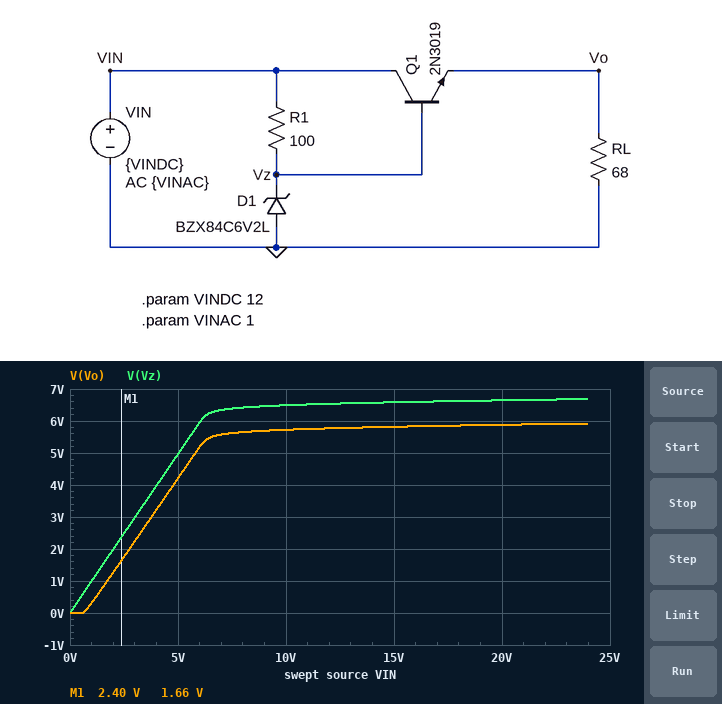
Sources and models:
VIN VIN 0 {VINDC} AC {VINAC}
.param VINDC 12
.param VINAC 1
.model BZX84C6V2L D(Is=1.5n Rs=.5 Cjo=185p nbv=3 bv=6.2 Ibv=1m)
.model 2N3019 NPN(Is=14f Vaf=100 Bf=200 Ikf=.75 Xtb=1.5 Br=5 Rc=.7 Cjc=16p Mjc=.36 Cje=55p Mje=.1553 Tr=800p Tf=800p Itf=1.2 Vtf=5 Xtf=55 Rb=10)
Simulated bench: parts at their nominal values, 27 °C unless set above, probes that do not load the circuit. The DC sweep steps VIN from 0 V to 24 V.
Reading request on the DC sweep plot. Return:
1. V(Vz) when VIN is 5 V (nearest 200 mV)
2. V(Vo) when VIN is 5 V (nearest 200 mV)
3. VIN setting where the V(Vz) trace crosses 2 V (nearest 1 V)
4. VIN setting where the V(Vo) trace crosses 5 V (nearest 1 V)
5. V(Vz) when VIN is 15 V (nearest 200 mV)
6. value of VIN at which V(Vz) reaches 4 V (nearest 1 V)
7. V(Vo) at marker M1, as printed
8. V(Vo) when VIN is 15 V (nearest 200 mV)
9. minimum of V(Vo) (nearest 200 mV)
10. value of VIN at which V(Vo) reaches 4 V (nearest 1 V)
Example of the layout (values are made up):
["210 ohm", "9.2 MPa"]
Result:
["5.0 V", "4.2 V", "2 V", "6 V", "6.6 V", "4 V", "1.66 V", "5.8 V", "0 V", "5 V"]
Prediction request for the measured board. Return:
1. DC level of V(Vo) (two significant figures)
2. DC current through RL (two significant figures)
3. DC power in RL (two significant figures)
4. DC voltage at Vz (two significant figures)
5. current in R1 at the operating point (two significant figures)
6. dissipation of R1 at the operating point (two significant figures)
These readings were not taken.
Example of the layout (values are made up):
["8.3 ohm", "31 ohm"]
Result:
["5.8 V", "85 mA", "490 mW", "6.5 V", "55 mA", "300 mW"]
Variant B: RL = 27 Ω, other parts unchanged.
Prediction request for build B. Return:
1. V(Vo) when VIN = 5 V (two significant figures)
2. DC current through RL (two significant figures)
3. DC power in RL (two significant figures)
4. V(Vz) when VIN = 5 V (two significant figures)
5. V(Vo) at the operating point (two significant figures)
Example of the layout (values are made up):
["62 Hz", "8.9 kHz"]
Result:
["4.1 V", "210 mA", "1.2 W", "4.9 V", "5.7 V"]
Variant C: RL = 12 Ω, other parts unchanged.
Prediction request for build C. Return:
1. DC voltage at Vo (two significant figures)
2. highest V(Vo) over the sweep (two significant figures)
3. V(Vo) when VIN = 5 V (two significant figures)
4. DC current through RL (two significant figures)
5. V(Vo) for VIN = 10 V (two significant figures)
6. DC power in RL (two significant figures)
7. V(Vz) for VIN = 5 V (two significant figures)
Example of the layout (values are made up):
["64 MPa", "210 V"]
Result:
["5.7 V", "5.8 V", "3.9 V", "470 mA", "5.6 V", "2.7 W", "4.8 V"]
